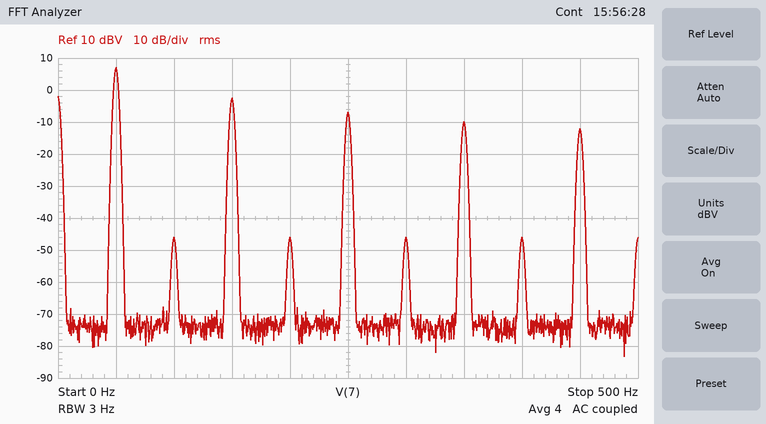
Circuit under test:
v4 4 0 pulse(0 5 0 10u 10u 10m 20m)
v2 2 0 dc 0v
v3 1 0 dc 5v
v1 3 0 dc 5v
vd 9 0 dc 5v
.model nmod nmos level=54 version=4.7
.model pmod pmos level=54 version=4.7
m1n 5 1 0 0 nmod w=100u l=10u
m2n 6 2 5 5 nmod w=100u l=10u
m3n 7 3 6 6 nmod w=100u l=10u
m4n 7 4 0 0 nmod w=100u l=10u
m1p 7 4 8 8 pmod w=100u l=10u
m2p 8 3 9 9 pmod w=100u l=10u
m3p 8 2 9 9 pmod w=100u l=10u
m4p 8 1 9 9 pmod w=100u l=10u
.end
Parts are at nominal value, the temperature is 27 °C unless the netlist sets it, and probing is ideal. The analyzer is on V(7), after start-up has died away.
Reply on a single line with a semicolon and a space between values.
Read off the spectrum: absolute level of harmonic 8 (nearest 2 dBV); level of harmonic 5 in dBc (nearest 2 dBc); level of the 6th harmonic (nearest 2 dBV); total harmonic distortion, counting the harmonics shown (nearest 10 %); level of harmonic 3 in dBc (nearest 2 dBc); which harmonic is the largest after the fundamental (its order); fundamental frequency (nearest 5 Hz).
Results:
-46 dBV; -14 dBc; -46 dBV; 40 %; -10 dBc; 3; 50 Hz
